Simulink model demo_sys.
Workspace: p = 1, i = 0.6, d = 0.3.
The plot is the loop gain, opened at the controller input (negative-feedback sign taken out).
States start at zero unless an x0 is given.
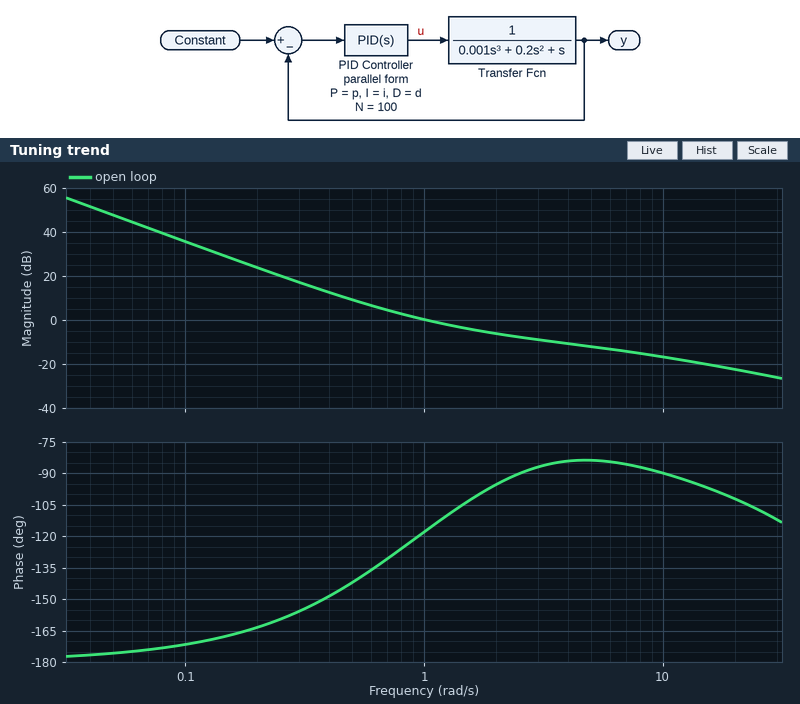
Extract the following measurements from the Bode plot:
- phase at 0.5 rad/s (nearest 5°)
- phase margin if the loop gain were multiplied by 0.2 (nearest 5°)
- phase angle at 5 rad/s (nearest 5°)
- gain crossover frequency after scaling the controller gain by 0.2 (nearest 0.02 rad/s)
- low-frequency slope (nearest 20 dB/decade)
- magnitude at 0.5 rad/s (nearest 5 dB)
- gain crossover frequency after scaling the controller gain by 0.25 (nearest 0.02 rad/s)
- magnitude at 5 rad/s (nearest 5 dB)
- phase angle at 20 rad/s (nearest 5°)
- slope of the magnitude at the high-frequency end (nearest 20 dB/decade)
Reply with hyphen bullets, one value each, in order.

- -140°
- 30°
- -85°
- 0.36 rad/s
- -40 dB/decade
- 10 dB
- 0.42 rad/s
- -10 dB
- -100°
- -20 dB/decade
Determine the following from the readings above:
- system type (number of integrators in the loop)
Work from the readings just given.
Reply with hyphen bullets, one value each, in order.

- 2
